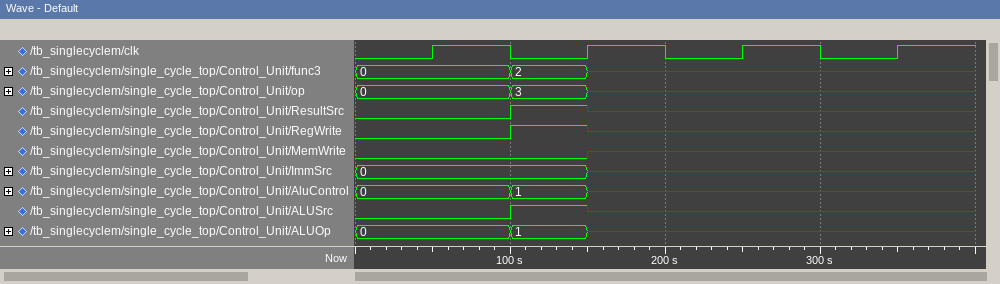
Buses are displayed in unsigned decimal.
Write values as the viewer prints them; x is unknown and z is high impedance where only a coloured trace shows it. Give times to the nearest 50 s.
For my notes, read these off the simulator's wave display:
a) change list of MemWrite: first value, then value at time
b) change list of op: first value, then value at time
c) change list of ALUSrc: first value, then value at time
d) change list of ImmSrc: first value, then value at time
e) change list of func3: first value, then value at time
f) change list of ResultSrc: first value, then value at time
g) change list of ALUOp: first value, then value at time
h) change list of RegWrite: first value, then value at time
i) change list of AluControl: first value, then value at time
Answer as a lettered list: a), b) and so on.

a) 0, x at 150 s
b) 0, 3 at 100 s, x at 150 s
c) 0, 1 at 100 s, x at 150 s
d) 0, x at 150 s
e) 0, 2 at 100 s, x at 150 s
f) 0, 1 at 100 s, x at 150 s
g) 0, 1 at 100 s, x at 150 s
h) 0, 1 at 100 s, x at 150 s
i) 0, 1 at 100 s, x at 150 s
